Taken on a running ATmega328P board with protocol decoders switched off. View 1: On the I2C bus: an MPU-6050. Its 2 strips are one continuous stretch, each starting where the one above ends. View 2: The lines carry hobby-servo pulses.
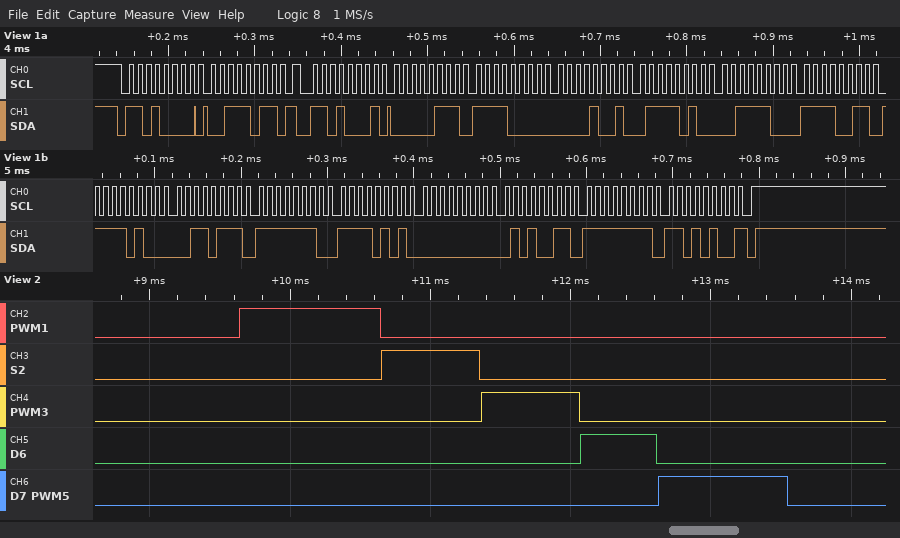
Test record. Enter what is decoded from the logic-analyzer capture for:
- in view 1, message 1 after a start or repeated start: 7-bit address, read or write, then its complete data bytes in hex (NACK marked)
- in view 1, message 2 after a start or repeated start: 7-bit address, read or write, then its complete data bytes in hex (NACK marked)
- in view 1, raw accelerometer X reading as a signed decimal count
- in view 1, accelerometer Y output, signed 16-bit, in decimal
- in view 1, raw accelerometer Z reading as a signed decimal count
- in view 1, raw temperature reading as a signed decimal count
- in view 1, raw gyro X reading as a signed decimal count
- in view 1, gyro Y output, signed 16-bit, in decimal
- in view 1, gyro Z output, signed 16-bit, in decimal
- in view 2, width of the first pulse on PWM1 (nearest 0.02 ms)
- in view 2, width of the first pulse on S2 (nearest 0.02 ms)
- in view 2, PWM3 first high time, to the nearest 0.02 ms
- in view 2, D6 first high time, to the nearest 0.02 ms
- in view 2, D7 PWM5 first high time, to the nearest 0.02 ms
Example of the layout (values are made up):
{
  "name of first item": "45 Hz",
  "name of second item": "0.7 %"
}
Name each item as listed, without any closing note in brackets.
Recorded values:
{
  "in view 1, message 1 after a start or repeated start: 7-bit address, read or write, then its complete data bytes in hex": "0x68 write: 3B",
  "in view 1, message 2 after a start or repeated start: 7-bit address, read or write, then its complete data bytes in hex": "0x68 read: 07 F0 09 7A 3C F3 F4 37 FE F5 00 53 FF D4 NACK",
  "in view 1, raw accelerometer X reading as a signed decimal count": "2032",
  "in view 1, accelerometer Y output, signed 16-bit, in decimal": "2426",
  "in view 1, raw accelerometer Z reading as a signed decimal count": "15603",
  "in view 1, raw temperature reading as a signed decimal count": "-3017",
  "in view 1, raw gyro X reading as a signed decimal count": "-267",
  "in view 1, gyro Y output, signed 16-bit, in decimal": "83",
  "in view 1, gyro Z output, signed 16-bit, in decimal": "-44",
  "in view 2, width of the first pulse on PWM1": "1.00 ms",
  "in view 2, width of the first pulse on S2": "0.70 ms",
  "in view 2, PWM3 first high time, to the nearest 0.02 ms": "0.70 ms",
  "in view 2, D6 first high time, to the nearest 0.02 ms": "0.54 ms",
  "in view 2, D7 PWM5 first high time, to the nearest 0.02 ms": "0.92 ms"
}
